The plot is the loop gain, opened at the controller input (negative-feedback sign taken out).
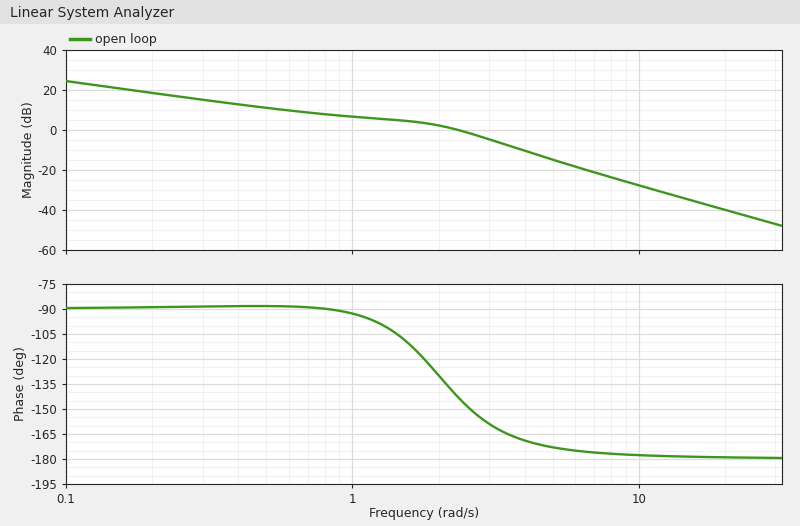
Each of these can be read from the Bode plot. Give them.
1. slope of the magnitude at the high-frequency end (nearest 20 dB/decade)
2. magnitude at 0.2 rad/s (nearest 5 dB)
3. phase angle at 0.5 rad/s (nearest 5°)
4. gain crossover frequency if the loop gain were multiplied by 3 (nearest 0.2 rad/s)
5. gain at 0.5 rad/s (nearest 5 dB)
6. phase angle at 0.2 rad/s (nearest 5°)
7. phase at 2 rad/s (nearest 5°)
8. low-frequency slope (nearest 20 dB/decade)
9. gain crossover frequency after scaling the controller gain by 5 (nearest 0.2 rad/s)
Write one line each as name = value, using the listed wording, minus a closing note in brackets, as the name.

slope of the magnitude at the high-frequency end = -40 dB/decade
magnitude at 0.2 rad/s = 20 dB
phase angle at 0.5 rad/s = -90°
gain crossover frequency if the loop gain were multiplied by 3 = 3.8 rad/s
gain at 0.5 rad/s = 10 dB
phase angle at 0.2 rad/s = -90°
phase at 2 rad/s = -130°
low-frequency slope = -20 dB/decade
gain crossover frequency after scaling the controller gain by 5 = 4.8 rad/s
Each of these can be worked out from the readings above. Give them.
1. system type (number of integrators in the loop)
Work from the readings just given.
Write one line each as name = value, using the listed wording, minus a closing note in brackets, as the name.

system type = 1
